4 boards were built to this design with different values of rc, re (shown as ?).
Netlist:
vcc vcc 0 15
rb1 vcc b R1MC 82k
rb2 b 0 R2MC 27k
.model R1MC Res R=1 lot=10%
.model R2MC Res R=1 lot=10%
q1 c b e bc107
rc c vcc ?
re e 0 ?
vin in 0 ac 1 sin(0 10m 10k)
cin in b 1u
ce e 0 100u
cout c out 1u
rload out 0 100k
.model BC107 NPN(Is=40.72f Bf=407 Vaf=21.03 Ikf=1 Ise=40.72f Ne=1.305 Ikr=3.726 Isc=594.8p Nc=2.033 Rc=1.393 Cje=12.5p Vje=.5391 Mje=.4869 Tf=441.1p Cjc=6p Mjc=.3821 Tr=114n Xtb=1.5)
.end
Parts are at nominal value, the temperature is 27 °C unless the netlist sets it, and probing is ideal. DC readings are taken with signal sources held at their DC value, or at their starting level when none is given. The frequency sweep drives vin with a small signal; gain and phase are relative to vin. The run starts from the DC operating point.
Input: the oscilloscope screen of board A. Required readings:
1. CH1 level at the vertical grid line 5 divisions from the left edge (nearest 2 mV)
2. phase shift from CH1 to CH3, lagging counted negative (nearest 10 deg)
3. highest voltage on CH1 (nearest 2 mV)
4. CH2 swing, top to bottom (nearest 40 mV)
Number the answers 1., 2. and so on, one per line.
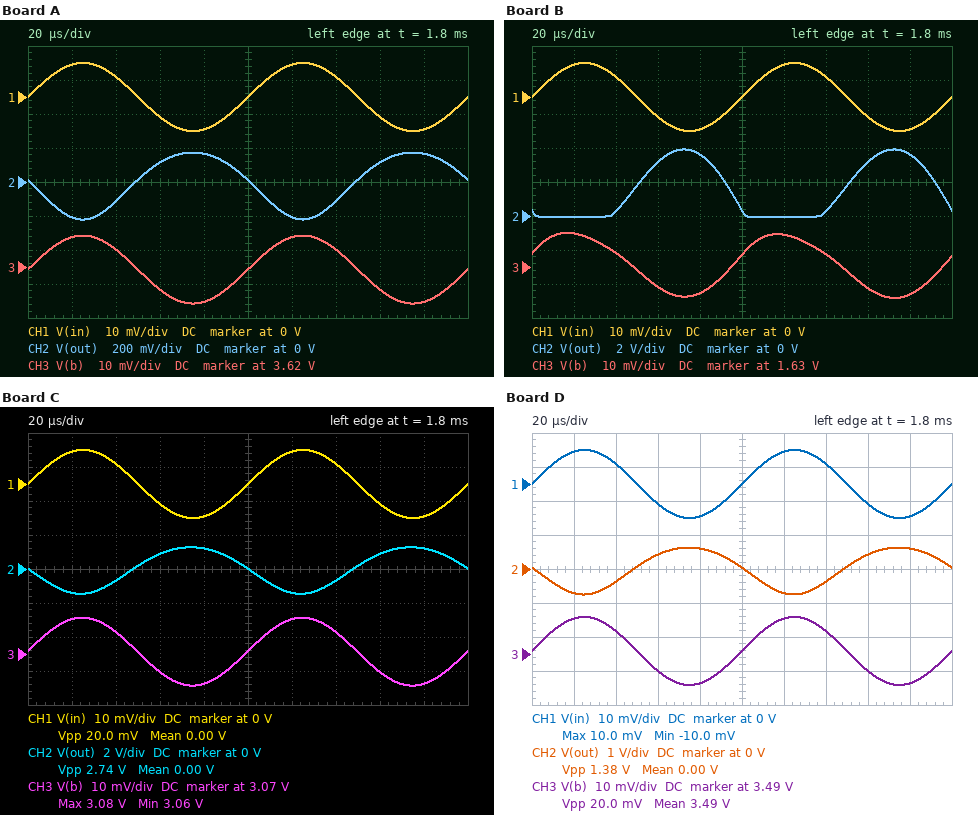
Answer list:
1. 0 V
2. 0 deg
3. 10 mV
4. 400 mV
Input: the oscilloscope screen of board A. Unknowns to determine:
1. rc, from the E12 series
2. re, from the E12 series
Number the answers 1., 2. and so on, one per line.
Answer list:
1. 470 Ω
2. 2.7 kΩ
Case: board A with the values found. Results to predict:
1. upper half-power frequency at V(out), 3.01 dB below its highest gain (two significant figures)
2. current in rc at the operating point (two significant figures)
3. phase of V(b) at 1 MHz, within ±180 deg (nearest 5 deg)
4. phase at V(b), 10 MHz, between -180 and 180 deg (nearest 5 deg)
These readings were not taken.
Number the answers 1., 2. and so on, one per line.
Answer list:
1. 160 MHz
2. 1.1 mA
3. 0 deg
4. 0 deg
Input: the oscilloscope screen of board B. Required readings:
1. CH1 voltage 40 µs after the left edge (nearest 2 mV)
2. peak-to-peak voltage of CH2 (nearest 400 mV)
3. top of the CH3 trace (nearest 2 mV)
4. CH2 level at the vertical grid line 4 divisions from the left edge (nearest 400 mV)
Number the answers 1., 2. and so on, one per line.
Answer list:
1. 6 mV
2. 4.0 V
3. 1.640 V
4. 3.6 V
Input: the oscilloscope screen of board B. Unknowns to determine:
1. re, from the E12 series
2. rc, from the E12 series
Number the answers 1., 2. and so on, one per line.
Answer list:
1. 270 Ω
2. 3.9 kΩ
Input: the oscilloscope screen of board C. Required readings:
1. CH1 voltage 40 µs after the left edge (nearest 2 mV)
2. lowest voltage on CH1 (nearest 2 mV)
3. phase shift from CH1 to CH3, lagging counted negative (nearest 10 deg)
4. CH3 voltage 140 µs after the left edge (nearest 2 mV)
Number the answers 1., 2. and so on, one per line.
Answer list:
1. 6 mV
2. -10 mV
3. 0 deg
4. 3.076 V
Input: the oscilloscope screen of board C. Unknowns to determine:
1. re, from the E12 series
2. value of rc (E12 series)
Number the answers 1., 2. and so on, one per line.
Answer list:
1. 270 Ω
2. 470 Ω
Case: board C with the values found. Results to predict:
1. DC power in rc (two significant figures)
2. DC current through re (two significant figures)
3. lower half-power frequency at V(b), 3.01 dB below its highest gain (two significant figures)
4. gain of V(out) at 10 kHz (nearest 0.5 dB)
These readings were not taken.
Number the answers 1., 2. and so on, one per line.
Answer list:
1. 37 mW
2. 8.9 mA
3. 26 Hz
4. 43.0 dB
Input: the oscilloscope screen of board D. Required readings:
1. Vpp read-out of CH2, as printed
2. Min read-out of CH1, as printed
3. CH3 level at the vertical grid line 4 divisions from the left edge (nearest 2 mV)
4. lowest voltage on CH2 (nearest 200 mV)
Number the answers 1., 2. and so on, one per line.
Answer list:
1. 1.38 V
2. -10.0 mV
3. 3.482 V
4. -800 mV
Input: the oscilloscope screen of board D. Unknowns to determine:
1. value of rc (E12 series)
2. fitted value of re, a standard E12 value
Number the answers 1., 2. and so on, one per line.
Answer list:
1. 680 Ω
2. 1 kΩ
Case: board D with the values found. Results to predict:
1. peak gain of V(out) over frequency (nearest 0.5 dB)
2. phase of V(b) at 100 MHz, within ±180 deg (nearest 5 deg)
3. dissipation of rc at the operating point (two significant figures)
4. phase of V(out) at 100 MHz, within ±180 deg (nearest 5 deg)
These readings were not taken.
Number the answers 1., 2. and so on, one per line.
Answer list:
1. 37.0 dB
2. 0 deg
3. 5.5 mW
4. 140 deg
